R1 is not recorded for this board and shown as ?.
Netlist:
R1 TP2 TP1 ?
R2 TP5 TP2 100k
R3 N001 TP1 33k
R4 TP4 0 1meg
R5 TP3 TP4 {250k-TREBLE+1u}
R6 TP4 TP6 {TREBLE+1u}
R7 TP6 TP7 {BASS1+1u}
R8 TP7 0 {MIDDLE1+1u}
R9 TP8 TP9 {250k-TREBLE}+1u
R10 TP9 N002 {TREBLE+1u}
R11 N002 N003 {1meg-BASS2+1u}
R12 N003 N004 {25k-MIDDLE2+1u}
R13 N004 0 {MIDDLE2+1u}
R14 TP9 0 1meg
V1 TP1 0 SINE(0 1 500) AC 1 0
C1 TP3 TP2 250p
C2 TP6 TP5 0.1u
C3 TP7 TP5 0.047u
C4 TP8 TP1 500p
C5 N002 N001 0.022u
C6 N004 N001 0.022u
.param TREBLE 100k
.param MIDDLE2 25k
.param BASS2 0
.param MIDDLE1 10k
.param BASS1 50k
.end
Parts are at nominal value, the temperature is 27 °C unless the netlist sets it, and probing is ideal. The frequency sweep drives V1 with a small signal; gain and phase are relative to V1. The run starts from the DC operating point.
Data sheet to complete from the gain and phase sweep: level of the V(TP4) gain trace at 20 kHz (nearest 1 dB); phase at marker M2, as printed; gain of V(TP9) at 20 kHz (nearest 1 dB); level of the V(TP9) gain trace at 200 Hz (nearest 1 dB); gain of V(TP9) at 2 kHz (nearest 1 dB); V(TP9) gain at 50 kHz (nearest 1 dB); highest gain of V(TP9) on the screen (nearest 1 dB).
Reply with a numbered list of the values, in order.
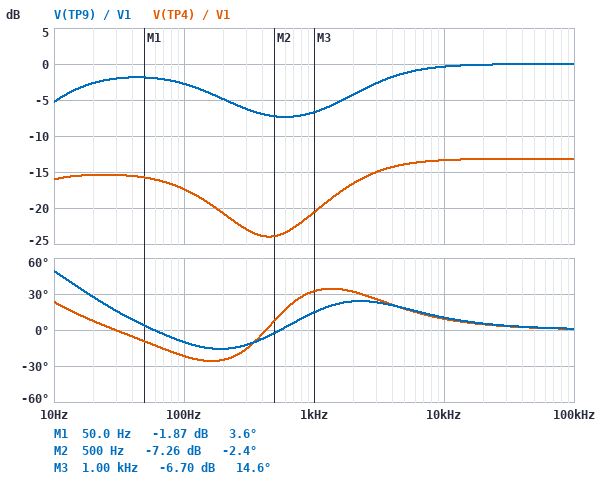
1. -13 dB
2. -2.4 deg
3. 0 dB
4. -5 dB
5. -4 dB
6. 0 dB
7. 0 dB
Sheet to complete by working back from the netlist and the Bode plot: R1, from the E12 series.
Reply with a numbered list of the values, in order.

1. 82 kΩ
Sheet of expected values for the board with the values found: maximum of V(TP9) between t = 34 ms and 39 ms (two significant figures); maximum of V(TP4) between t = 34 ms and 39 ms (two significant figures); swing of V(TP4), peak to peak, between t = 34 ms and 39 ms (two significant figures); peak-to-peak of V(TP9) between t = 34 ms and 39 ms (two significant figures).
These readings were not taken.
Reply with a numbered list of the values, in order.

1. 430 mV
2. 63 mV
3. 130 mV
4. 870 mV
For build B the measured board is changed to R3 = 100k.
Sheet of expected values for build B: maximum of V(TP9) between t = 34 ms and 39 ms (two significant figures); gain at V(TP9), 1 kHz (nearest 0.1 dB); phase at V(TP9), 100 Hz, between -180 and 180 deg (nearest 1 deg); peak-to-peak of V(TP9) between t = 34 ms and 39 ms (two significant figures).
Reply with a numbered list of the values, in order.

1. 230 mV
2. -9.4 dB
3. -26 deg
4. 460 mV
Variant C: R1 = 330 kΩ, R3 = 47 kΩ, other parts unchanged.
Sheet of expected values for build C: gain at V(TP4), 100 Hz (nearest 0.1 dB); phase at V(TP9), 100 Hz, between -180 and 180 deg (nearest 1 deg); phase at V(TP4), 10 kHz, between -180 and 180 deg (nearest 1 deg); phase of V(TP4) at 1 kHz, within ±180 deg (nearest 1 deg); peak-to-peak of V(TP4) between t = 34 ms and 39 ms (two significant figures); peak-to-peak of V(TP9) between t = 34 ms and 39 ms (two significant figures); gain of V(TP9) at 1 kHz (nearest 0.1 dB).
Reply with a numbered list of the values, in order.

1. -24.3 dB
2. -15 deg
3. 8 deg
4. 30 deg
5. 56 mV
6. 710 mV
7. -7.8 dB
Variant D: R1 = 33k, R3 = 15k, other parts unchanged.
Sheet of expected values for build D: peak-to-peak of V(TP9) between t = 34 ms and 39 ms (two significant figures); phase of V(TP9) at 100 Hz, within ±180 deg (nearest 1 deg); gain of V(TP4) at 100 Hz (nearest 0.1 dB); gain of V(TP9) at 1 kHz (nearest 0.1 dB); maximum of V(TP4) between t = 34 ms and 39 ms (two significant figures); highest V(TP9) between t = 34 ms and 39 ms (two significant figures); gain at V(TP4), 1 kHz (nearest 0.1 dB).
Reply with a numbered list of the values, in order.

1. 1.2 V
2. -2 deg
3. -15.0 dB
4. -4.3 dB
5. 85 mV
6. 610 mV
7. -18.0 dB
